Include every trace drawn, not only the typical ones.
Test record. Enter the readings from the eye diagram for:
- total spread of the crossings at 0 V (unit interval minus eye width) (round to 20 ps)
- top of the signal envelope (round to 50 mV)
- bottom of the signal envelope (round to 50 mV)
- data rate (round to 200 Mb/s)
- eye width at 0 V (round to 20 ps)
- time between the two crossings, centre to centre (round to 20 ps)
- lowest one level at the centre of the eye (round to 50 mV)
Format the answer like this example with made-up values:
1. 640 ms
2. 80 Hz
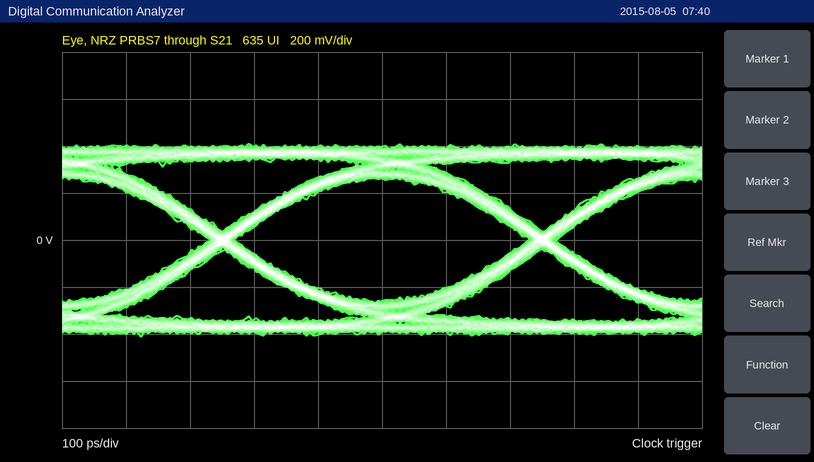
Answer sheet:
1. 40 ps
2. 400 mV
3. -400 mV
4. 2.0 Gb/s
5. 460 ps
6. 500 ps
7. 250 mV
